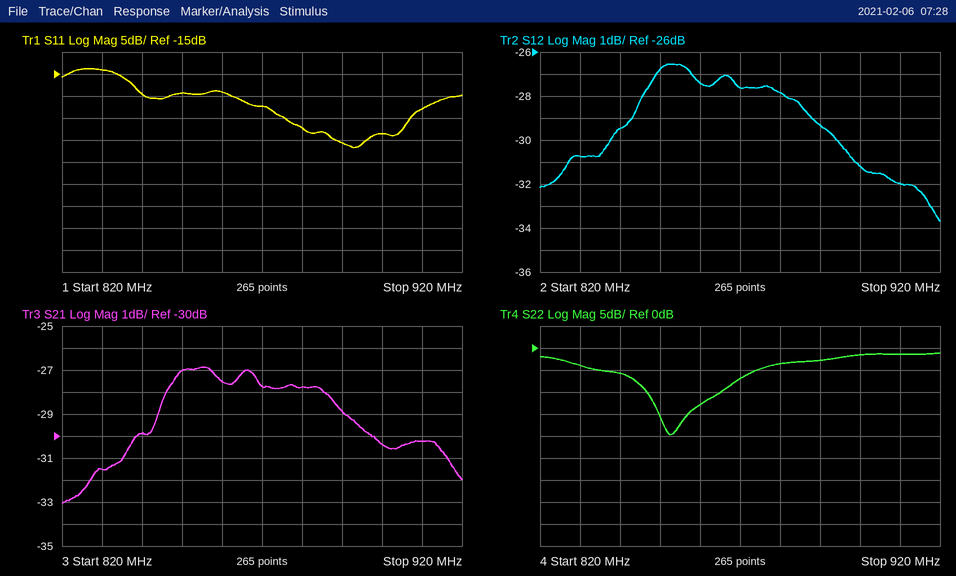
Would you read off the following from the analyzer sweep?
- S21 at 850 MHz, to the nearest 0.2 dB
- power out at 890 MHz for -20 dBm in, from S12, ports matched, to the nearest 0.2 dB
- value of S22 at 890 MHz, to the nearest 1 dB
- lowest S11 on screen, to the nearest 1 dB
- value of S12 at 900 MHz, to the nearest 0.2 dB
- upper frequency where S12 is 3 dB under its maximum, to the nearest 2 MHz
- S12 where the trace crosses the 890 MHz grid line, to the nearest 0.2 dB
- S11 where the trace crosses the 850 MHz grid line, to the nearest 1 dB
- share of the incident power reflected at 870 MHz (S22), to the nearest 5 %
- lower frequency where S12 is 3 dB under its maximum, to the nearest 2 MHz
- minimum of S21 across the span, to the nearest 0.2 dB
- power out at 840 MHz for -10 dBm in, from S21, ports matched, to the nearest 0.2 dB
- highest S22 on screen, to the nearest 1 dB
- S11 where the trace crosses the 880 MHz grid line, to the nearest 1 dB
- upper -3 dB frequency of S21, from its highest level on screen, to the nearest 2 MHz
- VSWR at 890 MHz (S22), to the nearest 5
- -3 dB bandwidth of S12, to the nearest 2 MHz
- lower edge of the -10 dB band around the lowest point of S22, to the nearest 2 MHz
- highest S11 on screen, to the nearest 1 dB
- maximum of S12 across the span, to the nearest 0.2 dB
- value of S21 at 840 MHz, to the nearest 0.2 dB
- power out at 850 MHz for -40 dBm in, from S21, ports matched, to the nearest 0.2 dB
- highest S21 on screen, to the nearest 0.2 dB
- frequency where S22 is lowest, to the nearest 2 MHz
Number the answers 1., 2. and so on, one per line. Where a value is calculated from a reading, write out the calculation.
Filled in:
1. -27.0 dB
2. -20 dBm + (-29.4 dB) = -49.4 dBm
3. -3 dB
4. -32 dB
5. -31.2 dB
6. 892 MHz
7. -29.4 dB
8. -19 dB
9. 10^(-7/10) ≈ 20 %
10. 840 MHz
11. -33.0 dB
12. -10 dBm + (-29.8 dB) = -39.8 dBm
13. -1 dB
14. -27 dB
15. 896 MHz
16. |Γ| = 10^(-3/20) = 0.7079; VSWR = (1 + 0.7079)/(1 − 0.7079) ≈ 5.85, so 5 to the nearest 5
17. 892 MHz − 840 MHz = 52 MHz
18. 846 MHz
19. -14 dB
20. -26.6 dB
21. -29.8 dB
22. -40 dBm + (-27.0 dB) = -67.0 dBm
23. -26.8 dB
24. 852 MHz
